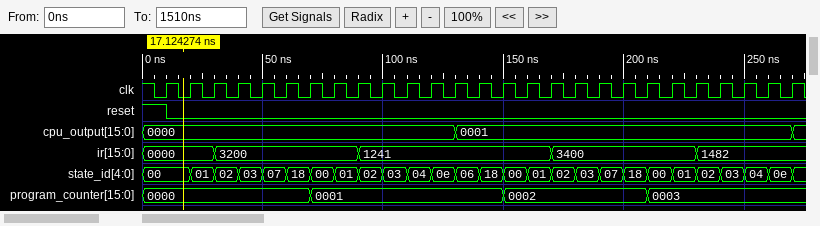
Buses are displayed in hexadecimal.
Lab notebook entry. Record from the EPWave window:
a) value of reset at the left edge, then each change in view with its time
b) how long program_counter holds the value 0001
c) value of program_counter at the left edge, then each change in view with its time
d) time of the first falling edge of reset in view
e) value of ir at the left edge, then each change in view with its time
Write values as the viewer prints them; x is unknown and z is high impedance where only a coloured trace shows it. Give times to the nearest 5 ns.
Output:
1, 0 at 10 ns
80 ns
0000, 0001 at 70 ns, 0002 at 150 ns, 0003 at 210 ns
10 ns
0000, 3200 at 30 ns, 1241 at 90 ns, 3400 at 170 ns, 1482 at 230 ns
